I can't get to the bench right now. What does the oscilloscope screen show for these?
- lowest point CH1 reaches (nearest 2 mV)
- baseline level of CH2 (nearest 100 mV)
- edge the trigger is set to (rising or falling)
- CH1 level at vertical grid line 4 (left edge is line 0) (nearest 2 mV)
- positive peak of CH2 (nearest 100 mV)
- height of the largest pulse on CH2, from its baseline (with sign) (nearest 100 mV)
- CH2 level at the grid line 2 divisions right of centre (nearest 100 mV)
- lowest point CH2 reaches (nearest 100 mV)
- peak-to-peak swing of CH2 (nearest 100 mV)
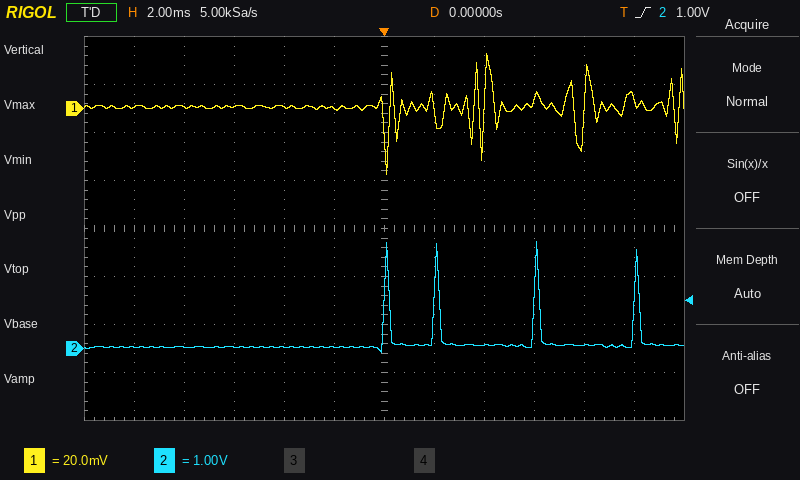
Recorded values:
-28 mV
0.0 V
rising
0 mV
2.2 V
+2.2 V
100 mV
-100 mV
2.3 V
